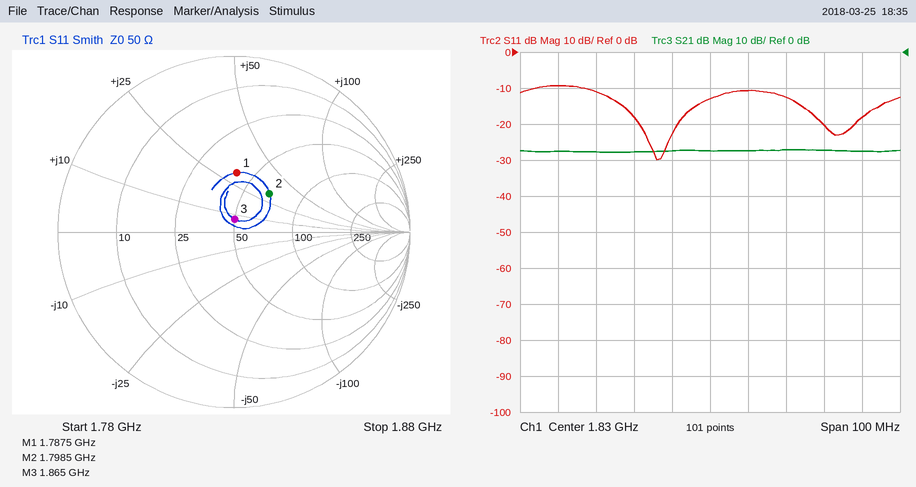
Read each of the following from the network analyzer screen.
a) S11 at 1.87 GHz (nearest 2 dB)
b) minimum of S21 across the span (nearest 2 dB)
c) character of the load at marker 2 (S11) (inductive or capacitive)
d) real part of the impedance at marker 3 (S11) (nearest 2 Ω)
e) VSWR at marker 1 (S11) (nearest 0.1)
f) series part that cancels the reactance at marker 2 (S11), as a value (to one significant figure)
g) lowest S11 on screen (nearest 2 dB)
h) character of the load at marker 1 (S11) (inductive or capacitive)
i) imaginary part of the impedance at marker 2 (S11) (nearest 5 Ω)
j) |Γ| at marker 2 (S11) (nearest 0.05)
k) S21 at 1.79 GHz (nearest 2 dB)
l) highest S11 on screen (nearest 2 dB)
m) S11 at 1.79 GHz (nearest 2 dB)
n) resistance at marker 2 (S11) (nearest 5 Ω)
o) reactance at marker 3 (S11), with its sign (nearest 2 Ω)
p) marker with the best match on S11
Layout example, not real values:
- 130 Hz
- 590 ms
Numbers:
- -18 dB
- -28 dB
- inductive
- 50 Ω
- 2.0
- 3 pF
- -30 dB
- inductive
- +30 Ω
- 0.30
- -28 dB
- -10 dB
- -10 dB
- 65 Ω
- +8 Ω
- marker 3
